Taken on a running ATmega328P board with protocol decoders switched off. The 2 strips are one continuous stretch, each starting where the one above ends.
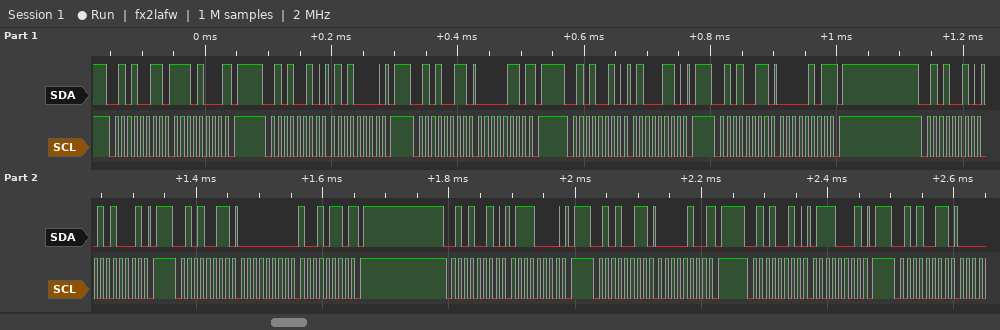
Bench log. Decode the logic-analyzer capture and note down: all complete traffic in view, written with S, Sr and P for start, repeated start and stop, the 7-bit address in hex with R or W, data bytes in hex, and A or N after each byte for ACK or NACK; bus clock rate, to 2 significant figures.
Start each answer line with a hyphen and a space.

- S 29R A E8 N P S 29W A 50 A P S 29R A 06 N P S 29W A 46 A P S 29R A 05 N P S 29W A 51 A P S 29R A 00 A 96 N P S 29W A 70 A P S 29R A 04 N P S 29W A 71 A P S 29R A
- 100 kHz
